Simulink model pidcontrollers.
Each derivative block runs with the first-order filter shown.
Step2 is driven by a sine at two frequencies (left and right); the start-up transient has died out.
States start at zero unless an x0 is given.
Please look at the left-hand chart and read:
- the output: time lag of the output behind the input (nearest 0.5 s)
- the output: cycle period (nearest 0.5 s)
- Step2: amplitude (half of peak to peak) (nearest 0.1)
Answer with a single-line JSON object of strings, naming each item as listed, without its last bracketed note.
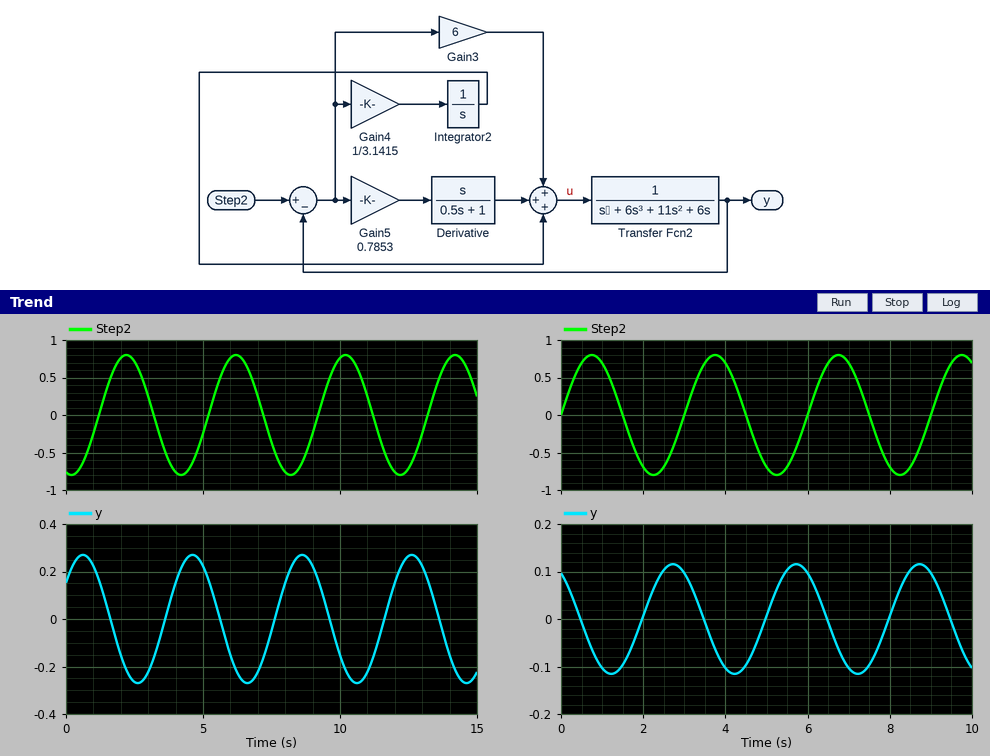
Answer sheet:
{"the output: time lag of the output behind the input": "2.5 s", "the output: cycle period": "4.0 s", "Step2: amplitude (half of peak to peak)": "0.8"}
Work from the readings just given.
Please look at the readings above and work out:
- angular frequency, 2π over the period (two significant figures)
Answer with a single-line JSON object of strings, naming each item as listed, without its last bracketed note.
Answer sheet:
{"angular frequency, 2π over the period": "1.6 rad/s"}
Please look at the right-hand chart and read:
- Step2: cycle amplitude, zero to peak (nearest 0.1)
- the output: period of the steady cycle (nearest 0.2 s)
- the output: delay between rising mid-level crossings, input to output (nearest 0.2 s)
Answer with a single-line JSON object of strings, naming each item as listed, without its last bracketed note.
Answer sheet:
{"Step2: cycle amplitude, zero to peak": "0.8", "the output: period of the steady cycle": "3.0 s", "the output: delay between rising mid-level crossings, input to output": "2.0 s"}
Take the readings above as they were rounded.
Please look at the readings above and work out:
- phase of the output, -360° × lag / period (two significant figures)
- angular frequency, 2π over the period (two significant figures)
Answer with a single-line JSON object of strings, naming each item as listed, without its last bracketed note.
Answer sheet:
{"phase of the output, -360° × lag / period": "-240°", "angular frequency, 2π over the period": "2.1 rad/s"}
